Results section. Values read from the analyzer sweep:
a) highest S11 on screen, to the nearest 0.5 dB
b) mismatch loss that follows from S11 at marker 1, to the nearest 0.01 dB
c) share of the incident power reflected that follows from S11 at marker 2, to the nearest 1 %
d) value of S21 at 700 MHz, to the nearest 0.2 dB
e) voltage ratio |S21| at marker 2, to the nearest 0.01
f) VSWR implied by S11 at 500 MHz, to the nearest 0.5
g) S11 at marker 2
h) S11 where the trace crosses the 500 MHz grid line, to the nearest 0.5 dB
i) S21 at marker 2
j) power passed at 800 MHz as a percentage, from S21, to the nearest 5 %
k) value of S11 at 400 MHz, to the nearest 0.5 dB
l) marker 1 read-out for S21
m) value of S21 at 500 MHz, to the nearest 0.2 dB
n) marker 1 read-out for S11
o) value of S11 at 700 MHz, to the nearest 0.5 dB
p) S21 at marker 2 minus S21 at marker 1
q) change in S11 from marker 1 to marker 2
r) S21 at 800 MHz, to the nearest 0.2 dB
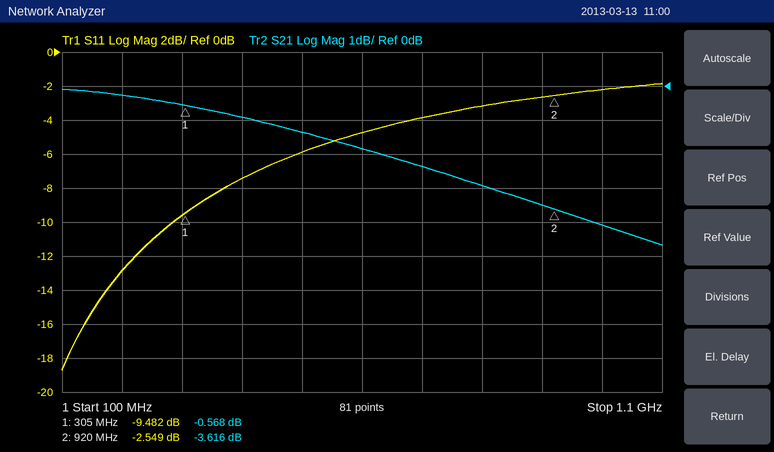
-2.0 dB
0.52 dB
56 %
-2.4 dB
0.66
3.0
-2.549 dB
-6.0 dB
-3.616 dB
50 %
-7.5 dB
-0.568 dB
-1.4 dB
-9.482 dB
-4.0 dB
-3.048 dB
6.933 dB
-3.0 dB
